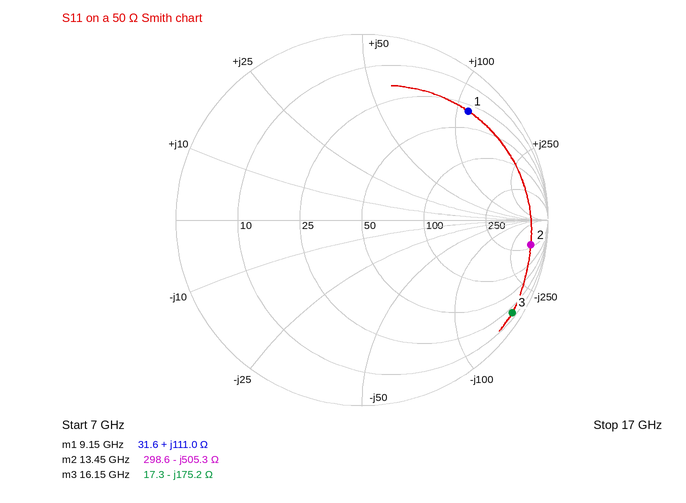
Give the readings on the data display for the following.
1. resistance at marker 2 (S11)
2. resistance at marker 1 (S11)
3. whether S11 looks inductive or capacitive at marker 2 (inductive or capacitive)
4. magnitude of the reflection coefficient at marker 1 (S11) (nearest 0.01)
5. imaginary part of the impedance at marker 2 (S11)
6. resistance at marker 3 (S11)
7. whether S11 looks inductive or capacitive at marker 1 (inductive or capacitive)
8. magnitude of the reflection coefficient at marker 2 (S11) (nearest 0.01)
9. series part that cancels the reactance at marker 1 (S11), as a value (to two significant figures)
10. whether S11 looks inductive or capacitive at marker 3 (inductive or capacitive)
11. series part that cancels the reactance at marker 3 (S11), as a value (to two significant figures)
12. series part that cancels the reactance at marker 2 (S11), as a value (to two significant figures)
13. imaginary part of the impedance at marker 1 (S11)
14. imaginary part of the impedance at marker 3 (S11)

298.6 Ω
31.6 Ω
capacitive
0.82
-505.3 Ω
17.3 Ω
inductive
0.92
160 fF
capacitive
1.7 nH
6.0 nH
+111.0 Ω
-175.2 Ω
